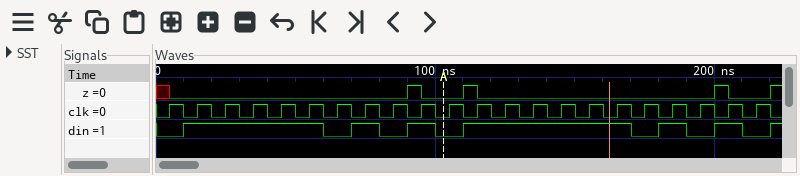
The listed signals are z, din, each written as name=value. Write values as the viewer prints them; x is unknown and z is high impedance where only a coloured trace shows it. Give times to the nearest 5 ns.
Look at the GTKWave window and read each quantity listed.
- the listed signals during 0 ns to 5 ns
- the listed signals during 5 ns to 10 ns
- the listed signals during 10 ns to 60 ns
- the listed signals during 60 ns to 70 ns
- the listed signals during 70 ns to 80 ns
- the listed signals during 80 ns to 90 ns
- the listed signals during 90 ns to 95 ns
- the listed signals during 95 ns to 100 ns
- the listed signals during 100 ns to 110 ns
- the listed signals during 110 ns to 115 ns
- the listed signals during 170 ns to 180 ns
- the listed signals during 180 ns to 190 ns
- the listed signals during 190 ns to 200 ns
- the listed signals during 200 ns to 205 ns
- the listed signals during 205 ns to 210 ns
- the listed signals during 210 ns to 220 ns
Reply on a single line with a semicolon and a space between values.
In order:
z=x, din=0; z=0, din=0; z=0, din=1; z=0, din=0; z=0, din=1; z=0, din=0; z=1, din=1; z=0, din=1; z=0, din=0; z=1, din=1; z=0, din=0; z=0, din=1; z=0, din=0; z=1, din=1; z=0, din=1; z=0, din=0
